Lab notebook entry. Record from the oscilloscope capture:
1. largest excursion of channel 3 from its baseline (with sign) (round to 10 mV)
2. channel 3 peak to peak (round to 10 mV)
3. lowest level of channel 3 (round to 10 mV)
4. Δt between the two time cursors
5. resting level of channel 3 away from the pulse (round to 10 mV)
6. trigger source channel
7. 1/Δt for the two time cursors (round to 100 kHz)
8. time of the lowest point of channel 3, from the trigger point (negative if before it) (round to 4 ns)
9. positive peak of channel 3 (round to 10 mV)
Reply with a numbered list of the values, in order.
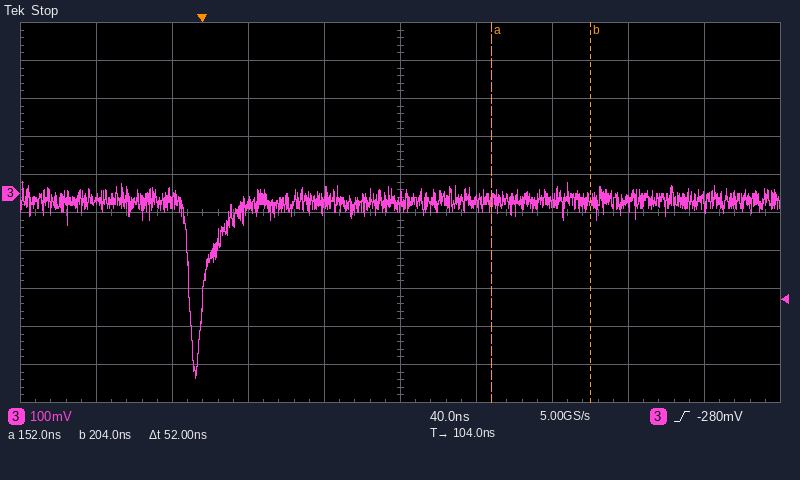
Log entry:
1. -470 mV
2. 520 mV
3. -490 mV
4. 52 ns
5. -20 mV
6. channel 3
7. 19.2 MHz
8. -4 ns
9. 30 mV
